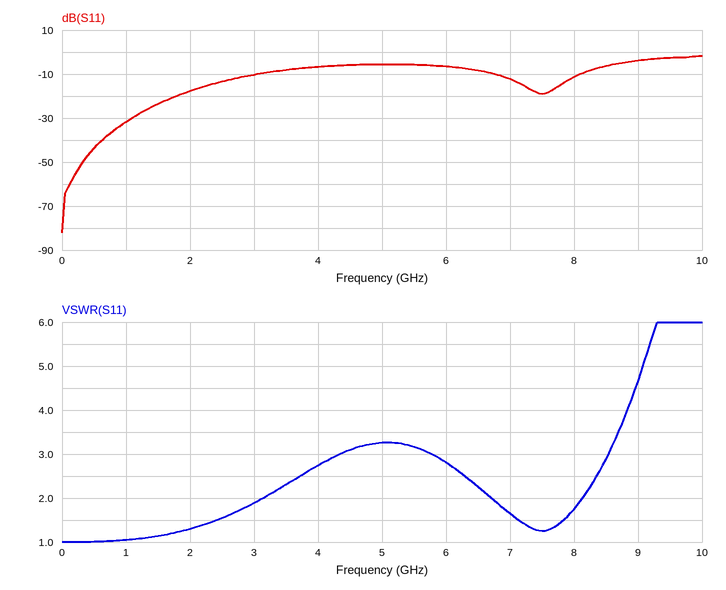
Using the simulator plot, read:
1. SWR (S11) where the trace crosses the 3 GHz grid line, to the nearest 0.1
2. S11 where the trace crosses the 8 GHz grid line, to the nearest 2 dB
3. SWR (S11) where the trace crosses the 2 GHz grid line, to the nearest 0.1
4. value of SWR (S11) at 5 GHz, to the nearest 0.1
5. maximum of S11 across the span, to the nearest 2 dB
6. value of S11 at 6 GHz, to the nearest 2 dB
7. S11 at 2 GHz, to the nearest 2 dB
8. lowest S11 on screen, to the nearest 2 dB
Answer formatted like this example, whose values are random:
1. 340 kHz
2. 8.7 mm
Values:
1. 1.9
2. -12 dB
3. 1.3
4. 3.3
5. -2 dB
6. -6 dB
7. -18 dB
8. -82 dB
